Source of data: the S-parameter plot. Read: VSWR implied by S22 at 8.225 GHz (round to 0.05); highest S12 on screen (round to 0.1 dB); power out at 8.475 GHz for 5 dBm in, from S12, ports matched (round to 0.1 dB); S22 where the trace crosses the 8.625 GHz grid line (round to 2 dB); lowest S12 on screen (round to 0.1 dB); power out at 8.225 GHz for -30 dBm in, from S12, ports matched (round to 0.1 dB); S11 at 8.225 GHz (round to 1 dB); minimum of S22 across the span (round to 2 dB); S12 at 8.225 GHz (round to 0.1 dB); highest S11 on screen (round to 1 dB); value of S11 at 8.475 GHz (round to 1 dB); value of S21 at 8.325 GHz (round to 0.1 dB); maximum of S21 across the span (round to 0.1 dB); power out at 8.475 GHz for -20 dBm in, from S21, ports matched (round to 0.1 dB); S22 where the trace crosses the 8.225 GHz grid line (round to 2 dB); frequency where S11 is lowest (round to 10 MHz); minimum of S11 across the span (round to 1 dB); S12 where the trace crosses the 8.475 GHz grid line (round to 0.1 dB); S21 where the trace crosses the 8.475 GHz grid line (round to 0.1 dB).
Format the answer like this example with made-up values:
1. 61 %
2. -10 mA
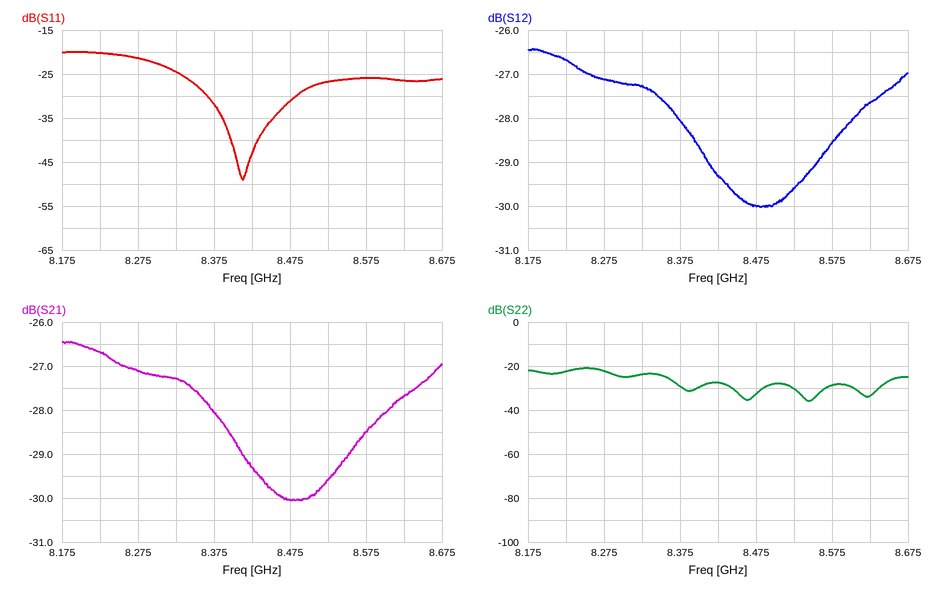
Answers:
1. 1.15
2. -26.4 dB
3. -25.0 dBm
4. -34 dB
5. -30.0 dB
6. -56.7 dBm
7. -20 dB
8. -36 dB
9. -26.7 dB
10. -20 dB
11. -31 dB
12. -27.3 dB
13. -26.4 dB
14. -50.0 dBm
15. -22 dB
16. 8.41 GHz
17. -49 dB
18. -30.0 dB
19. -30.0 dB
